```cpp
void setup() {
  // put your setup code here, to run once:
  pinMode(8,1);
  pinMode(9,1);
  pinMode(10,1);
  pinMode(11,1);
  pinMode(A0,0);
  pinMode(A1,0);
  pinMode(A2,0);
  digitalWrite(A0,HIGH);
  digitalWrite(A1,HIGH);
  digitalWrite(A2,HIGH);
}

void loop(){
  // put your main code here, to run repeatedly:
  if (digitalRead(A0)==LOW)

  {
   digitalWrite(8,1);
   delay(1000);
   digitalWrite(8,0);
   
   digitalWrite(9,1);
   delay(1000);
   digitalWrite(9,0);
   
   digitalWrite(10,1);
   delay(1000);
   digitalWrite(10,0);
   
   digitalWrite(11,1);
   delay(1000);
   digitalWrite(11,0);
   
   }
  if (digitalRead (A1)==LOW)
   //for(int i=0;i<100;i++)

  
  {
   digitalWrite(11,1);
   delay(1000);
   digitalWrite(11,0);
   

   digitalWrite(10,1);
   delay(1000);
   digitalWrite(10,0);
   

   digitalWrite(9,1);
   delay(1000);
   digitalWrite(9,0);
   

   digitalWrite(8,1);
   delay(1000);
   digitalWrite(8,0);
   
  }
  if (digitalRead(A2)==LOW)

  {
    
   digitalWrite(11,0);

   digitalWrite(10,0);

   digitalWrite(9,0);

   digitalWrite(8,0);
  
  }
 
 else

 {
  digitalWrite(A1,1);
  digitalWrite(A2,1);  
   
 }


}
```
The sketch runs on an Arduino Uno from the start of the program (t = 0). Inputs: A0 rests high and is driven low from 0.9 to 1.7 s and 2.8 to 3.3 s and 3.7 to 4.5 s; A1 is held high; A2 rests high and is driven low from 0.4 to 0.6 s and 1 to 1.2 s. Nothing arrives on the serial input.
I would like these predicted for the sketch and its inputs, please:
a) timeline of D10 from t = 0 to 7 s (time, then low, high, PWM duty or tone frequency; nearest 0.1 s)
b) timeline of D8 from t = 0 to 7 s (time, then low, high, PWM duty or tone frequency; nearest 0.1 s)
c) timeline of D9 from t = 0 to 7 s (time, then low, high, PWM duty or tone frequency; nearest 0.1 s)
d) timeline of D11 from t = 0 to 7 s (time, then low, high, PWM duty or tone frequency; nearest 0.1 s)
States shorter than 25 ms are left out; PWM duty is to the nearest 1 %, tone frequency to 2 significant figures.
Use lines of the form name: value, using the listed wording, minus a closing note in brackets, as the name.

timeline of D10 from t = 0 to 7 s: 0 s low; 2.9 s high; 3.9 s low
timeline of D8 from t = 0 to 7 s: 0 s low; 0.9 s high; 1.9 s low
timeline of D9 from t = 0 to 7 s: 0 s low; 1.9 s high; 2.9 s low
timeline of D11 from t = 0 to 7 s: 0 s low; 3.9 s high; 4.9 s low
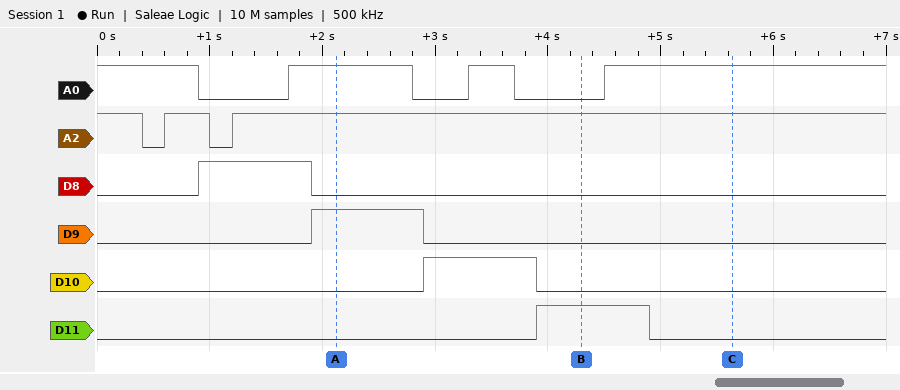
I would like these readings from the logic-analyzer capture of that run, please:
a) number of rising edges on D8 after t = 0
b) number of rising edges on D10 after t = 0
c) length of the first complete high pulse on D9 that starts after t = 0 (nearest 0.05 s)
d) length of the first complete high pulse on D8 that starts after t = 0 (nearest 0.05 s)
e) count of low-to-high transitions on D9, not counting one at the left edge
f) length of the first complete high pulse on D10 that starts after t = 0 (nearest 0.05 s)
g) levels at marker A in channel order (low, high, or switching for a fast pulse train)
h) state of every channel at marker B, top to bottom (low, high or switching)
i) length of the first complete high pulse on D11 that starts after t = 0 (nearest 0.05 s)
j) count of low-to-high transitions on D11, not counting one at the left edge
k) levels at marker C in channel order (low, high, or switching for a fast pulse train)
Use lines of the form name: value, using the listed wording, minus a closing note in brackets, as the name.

number of rising edges on D8 after t = 0: 1
number of rising edges on D10 after t = 0: 1
length of the first complete high pulse on D9 that starts after t = 0: 1.00 s
length of the first complete high pulse on D8 that starts after t = 0: 1.00 s
count of low-to-high transitions on D9, not counting one at the left edge: 1
length of the first complete high pulse on D10 that starts after t = 0: 1.00 s
levels at marker A in channel order: A0 high, A2 high, D8 low, D9 high, D10 low, D11 low
state of every channel at marker B, top to bottom: A0 low, A2 high, D8 low, D9 low, D10 low, D11 high
length of the first complete high pulse on D11 that starts after t = 0: 1.00 s
count of low-to-high transitions on D11, not counting one at the left edge: 1
levels at marker C in channel order: A0 high, A2 high, D8 low, D9 low, D10 low, D11 low
